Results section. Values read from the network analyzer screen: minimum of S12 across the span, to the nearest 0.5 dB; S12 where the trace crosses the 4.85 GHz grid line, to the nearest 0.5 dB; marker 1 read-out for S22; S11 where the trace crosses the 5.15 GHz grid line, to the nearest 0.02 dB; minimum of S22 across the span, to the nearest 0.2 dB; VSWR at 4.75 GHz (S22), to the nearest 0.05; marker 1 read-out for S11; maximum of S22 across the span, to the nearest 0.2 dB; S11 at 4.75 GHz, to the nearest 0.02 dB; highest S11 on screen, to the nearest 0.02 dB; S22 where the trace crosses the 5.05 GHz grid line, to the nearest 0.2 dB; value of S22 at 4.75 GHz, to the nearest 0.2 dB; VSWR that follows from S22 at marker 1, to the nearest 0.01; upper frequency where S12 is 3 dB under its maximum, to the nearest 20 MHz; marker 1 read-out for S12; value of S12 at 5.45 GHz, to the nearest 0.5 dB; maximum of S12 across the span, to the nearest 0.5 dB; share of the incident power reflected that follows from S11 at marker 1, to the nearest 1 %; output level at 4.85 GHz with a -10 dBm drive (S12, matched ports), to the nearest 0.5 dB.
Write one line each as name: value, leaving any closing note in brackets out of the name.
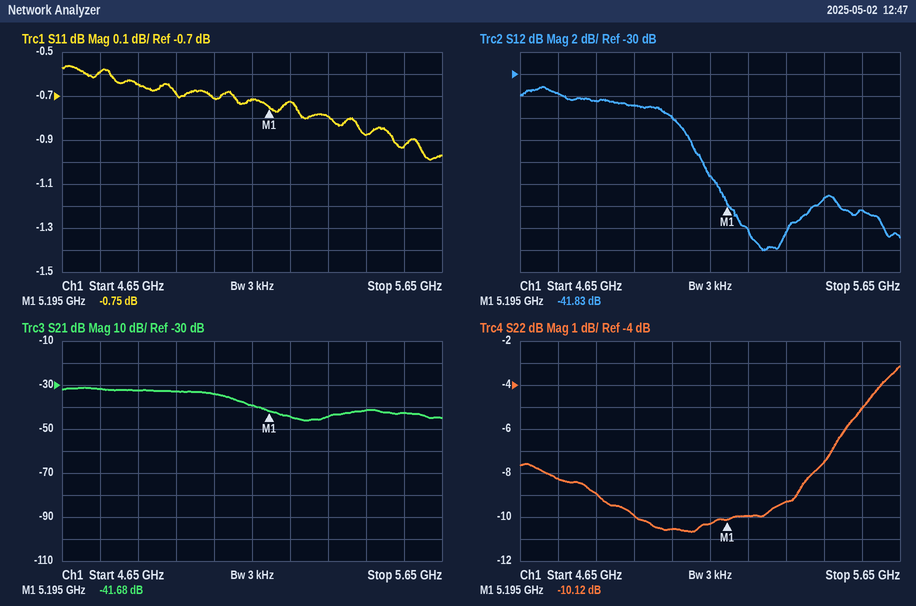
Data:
minimum of S12 across the span, to the nearest 0.5 dB: -46.0 dB
S12 where the trace crosses the 4.85 GHz grid line, to the nearest 0.5 dB: -32.5 dB
marker 1 read-out for S22: -10.12 dB
S11 where the trace crosses the 5.15 GHz grid line, to the nearest 0.02 dB: -0.72 dB
minimum of S22 across the span, to the nearest 0.2 dB: -10.6 dB
VSWR at 4.75 GHz (S22), to the nearest 0.05: 2.25
marker 1 read-out for S11: -0.75 dB
maximum of S22 across the span, to the nearest 0.2 dB: -3.2 dB
S11 at 4.75 GHz, to the nearest 0.02 dB: -0.60 dB
highest S11 on screen, to the nearest 0.02 dB: -0.56 dB
S22 where the trace crosses the 5.05 GHz grid line, to the nearest 0.2 dB: -10.6 dB
value of S22 at 4.75 GHz, to the nearest 0.2 dB: -8.2 dB
VSWR that follows from S22 at marker 1, to the nearest 0.01: 1.91
upper frequency where S12 is 3 dB under its maximum, to the nearest 20 MHz: 5.06 GHz
marker 1 read-out for S12: -41.83 dB
value of S12 at 5.45 GHz, to the nearest 0.5 dB: -41.5 dB
maximum of S12 across the span, to the nearest 0.5 dB: -31.0 dB
share of the incident power reflected that follows from S11 at marker 1, to the nearest 1 %: 84 %
output level at 4.85 GHz with a -10 dBm drive (S12, matched ports), to the nearest 0.5 dB: -42.5 dBm
